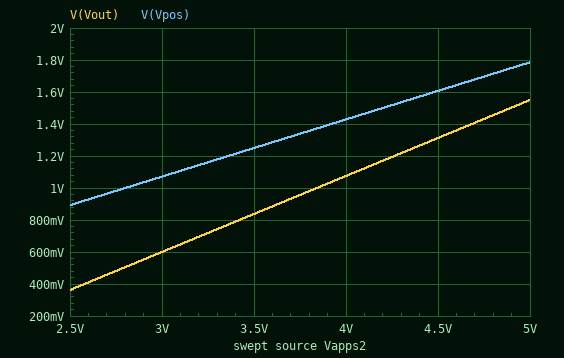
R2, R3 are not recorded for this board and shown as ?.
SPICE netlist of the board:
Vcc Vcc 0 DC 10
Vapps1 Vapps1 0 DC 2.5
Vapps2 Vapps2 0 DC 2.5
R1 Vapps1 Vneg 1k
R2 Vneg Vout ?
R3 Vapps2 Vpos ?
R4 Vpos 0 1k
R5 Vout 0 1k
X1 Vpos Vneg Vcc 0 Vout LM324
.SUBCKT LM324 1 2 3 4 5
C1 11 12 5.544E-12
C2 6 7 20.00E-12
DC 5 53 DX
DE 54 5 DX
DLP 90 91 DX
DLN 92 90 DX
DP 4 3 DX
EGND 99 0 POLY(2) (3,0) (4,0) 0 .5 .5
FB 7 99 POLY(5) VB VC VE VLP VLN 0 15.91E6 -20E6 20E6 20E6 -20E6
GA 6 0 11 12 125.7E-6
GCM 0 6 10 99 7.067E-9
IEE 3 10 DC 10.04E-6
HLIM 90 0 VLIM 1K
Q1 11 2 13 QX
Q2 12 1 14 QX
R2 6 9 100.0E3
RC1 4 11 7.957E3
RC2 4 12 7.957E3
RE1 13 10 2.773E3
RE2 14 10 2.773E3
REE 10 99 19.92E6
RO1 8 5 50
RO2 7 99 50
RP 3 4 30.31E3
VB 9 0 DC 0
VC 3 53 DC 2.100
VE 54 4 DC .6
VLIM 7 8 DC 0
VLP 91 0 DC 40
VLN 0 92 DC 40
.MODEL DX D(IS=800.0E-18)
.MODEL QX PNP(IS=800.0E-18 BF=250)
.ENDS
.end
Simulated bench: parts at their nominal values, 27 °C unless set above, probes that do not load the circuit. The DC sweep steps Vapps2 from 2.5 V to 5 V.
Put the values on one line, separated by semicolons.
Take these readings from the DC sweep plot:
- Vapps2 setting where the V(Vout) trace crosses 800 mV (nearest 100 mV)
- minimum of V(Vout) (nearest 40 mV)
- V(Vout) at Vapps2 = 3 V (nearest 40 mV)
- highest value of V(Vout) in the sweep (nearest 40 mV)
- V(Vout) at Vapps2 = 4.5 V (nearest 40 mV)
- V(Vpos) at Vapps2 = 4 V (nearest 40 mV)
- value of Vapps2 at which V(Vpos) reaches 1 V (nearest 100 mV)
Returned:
3.4 V; 360 mV; 600 mV; 1.56 V; 1.32 V; 1.44 V; 2.8 V
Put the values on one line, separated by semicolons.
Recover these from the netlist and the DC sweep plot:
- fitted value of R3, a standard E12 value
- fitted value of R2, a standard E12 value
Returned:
1.8 kΩ; 330 Ω
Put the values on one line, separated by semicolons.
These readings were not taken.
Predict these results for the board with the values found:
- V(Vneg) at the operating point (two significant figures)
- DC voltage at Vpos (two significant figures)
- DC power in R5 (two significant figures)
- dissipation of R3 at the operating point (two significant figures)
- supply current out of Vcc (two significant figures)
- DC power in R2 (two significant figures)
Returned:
890 mV; 890 mV; 130 µW; 1.4 mW; 340 µA; 850 µW
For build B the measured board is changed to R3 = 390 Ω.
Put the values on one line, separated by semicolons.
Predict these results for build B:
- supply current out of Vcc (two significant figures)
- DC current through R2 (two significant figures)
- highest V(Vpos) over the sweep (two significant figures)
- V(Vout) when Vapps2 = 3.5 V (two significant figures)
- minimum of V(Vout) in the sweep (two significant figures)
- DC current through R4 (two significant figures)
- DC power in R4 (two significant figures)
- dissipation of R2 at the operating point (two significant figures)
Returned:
340 µA; 700 µA; 3.6 V; 2.5 V; 1.6 V; 1.8 mA; 3.2 mW; 160 µW
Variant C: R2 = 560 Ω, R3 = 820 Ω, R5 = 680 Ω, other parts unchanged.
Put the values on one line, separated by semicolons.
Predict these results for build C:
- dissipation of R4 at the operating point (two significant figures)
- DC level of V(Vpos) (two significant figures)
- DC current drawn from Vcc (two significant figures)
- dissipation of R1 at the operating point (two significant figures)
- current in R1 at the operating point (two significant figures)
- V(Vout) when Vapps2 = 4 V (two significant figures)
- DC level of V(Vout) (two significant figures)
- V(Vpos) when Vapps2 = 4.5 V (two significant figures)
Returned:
1.9 mW; 1.4 V; 340 µA; 1.3 mW; 1.1 mA; 2.0 V; 740 mV; 2.5 V
